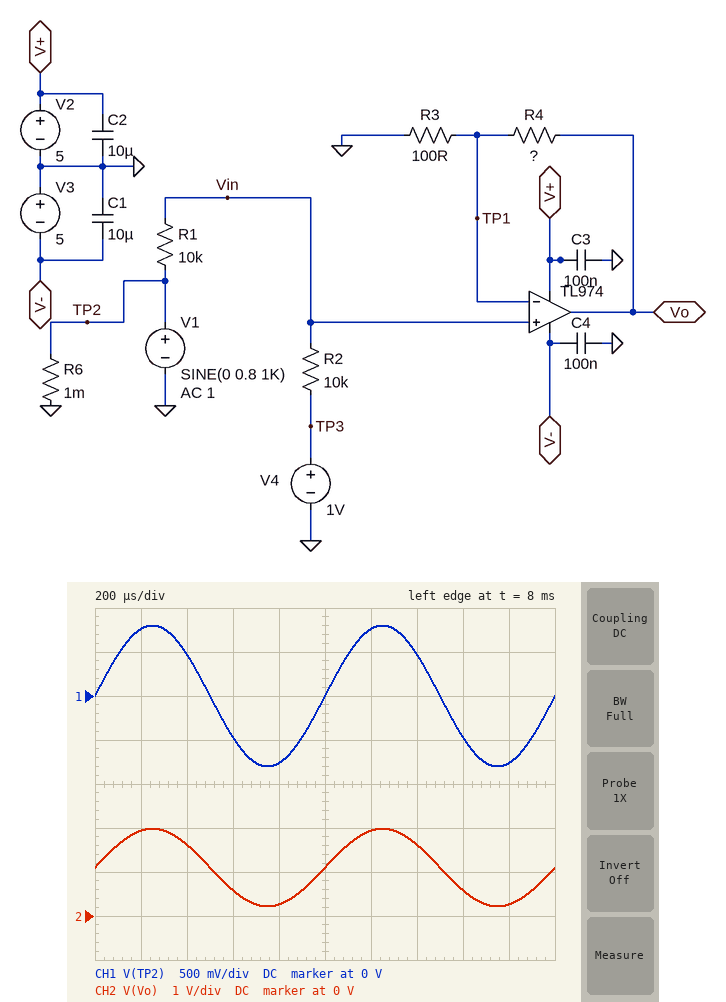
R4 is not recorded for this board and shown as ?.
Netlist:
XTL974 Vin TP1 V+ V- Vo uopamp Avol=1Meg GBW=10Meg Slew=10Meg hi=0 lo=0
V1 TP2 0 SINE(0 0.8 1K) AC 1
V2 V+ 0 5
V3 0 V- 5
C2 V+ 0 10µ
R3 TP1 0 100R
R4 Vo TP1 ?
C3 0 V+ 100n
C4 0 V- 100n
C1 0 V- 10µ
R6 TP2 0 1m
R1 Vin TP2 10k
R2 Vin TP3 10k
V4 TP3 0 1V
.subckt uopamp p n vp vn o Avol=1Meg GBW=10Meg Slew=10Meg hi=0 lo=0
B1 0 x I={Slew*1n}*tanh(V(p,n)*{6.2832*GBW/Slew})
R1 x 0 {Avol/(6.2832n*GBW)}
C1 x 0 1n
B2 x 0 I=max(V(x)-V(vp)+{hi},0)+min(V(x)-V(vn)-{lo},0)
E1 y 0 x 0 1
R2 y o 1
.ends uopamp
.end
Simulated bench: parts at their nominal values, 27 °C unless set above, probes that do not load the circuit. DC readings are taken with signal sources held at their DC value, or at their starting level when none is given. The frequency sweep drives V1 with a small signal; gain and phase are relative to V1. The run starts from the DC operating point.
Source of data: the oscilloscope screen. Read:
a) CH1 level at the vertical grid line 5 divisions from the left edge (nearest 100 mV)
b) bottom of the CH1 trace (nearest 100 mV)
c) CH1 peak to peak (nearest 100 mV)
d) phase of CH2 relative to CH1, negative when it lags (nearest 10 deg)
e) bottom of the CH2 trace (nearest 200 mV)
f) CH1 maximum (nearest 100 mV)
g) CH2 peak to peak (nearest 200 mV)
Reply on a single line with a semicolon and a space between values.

0 V; -800 mV; 1.6 V; 0 deg; 200 mV; 800 mV; 1.8 V
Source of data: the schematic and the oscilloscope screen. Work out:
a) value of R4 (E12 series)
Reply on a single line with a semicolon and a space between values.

120 Ω
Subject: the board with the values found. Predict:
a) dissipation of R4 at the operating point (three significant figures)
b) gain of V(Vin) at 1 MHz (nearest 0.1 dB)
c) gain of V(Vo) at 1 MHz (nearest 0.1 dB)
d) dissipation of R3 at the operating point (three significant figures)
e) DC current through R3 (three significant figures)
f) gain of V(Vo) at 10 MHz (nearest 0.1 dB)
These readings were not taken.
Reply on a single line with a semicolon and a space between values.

3.00 mW; -6.0 dB; 0.6 dB; 2.50 mW; 5.00 mA; -6.9 dB
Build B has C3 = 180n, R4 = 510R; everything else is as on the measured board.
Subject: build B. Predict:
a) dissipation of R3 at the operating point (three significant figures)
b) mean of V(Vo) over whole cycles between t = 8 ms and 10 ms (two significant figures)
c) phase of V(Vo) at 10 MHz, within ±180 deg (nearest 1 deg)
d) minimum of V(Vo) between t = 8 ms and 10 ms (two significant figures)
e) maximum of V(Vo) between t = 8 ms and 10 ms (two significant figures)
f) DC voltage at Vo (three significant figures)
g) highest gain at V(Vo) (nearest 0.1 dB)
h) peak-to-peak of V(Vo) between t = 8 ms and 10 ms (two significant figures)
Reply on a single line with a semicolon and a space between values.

2.50 mW; 3.0 V; -81 deg; 610 mV; 5.0 V; 3.05 V; 9.7 dB; 4.4 V
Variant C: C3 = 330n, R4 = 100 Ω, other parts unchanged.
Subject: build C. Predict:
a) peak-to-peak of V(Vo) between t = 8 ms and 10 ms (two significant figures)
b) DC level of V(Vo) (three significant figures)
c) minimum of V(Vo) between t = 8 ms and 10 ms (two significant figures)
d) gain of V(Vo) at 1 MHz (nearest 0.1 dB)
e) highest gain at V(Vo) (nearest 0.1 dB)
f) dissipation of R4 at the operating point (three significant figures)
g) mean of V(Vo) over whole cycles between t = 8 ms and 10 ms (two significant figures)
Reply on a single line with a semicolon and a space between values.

1.6 V; 1.00 V; 200 mV; -0.2 dB; 0 dB; 2.50 mW; 1.0 V
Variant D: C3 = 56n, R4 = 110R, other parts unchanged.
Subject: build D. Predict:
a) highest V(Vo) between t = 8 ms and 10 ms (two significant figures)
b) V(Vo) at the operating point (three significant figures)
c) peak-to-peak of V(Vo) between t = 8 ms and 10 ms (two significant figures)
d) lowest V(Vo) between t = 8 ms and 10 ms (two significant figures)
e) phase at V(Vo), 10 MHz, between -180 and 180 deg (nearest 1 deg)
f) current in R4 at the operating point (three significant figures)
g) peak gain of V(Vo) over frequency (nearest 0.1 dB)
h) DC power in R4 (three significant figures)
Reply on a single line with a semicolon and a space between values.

1.9 V; 1.05 V; 1.7 V; 210 mV; -65 deg; 5.00 mA; 0.4 dB; 2.75 mW
